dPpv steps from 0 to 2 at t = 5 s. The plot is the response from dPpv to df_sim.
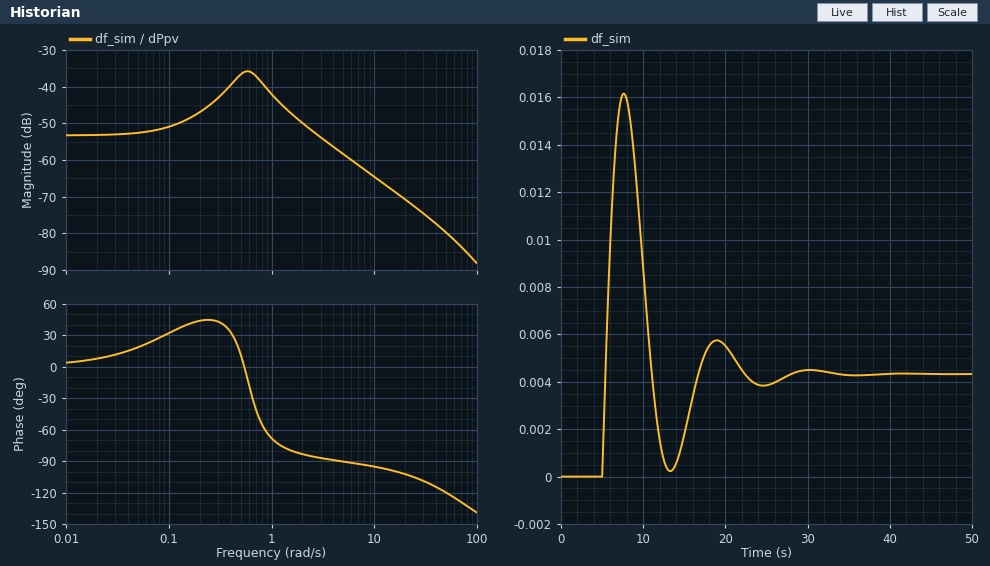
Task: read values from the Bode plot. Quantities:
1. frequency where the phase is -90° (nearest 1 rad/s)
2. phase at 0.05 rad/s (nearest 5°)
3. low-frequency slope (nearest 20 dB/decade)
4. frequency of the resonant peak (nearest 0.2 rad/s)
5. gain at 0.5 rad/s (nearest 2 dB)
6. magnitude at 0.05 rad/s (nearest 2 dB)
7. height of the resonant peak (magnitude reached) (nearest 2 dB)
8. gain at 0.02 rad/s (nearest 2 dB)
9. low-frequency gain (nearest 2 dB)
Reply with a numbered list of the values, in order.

1. 5 rad/s
2. 20°
3. 0 dB/decade
4. 0.6 rad/s
5. -36 dB
6. -52 dB
7. -36 dB
8. -54 dB
9. -54 dB
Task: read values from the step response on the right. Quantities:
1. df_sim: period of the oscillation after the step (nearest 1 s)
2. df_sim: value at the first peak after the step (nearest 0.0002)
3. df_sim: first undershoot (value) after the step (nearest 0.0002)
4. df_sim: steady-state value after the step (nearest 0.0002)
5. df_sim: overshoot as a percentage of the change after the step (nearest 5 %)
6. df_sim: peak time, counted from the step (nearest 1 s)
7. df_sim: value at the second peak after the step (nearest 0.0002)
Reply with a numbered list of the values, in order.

1. 11 s
2. 0.0162
3. 0.0002
4. 0.0044
5. 275 %
6. 3 s
7. 0.0058
